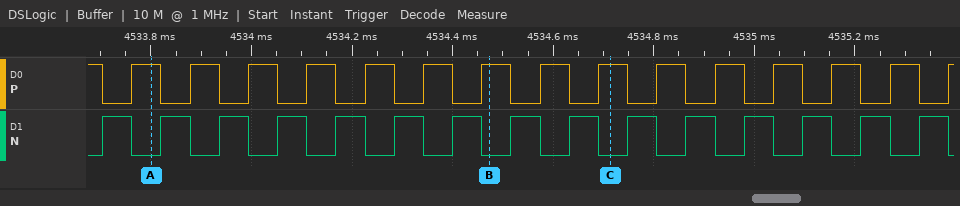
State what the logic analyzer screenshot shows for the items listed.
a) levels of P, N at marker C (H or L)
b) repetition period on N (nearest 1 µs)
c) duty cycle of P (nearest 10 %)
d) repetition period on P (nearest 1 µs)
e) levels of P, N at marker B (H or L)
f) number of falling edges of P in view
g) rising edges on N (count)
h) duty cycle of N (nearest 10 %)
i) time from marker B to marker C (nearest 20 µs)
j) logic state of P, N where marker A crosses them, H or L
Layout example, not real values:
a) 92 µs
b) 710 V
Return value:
a) P=H, N=L
b) 116 µs
c) 50 %
d) 116 µs
e) P=H, N=L
f) 15
g) 15
h) 50 %
i) 240 µs
j) P=H, N=L
